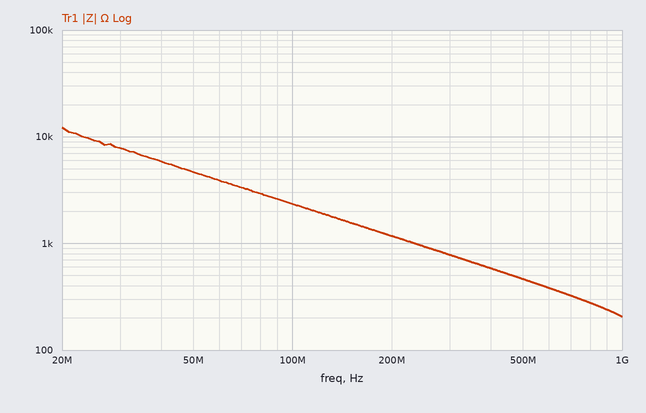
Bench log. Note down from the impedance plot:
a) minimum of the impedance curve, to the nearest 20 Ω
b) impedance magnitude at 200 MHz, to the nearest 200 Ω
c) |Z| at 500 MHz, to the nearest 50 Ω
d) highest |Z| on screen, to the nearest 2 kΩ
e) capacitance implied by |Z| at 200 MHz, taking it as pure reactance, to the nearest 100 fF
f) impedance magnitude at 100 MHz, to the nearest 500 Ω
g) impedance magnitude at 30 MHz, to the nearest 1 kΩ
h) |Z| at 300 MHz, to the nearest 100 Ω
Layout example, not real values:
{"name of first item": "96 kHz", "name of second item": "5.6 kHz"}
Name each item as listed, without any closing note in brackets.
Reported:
{"minimum of the impedance curve, to the nearest 20 Ω": "200 Ω", "impedance magnitude at 200 MHz, to the nearest 200 Ω": "1.2 kΩ", "|Z| at 500 MHz, to the nearest 50 Ω": "450 Ω", "highest |Z| on screen, to the nearest 2 kΩ": "12 kΩ", "capacitance implied by |Z| at 200 MHz, taking it as pure reactance, to the nearest 100 fF": "700 fF", "impedance magnitude at 100 MHz, to the nearest 500 Ω": "2.5 kΩ", "impedance magnitude at 30 MHz, to the nearest 1 kΩ": "8 kΩ", "|Z| at 300 MHz, to the nearest 100 Ω": "800 Ω"}
